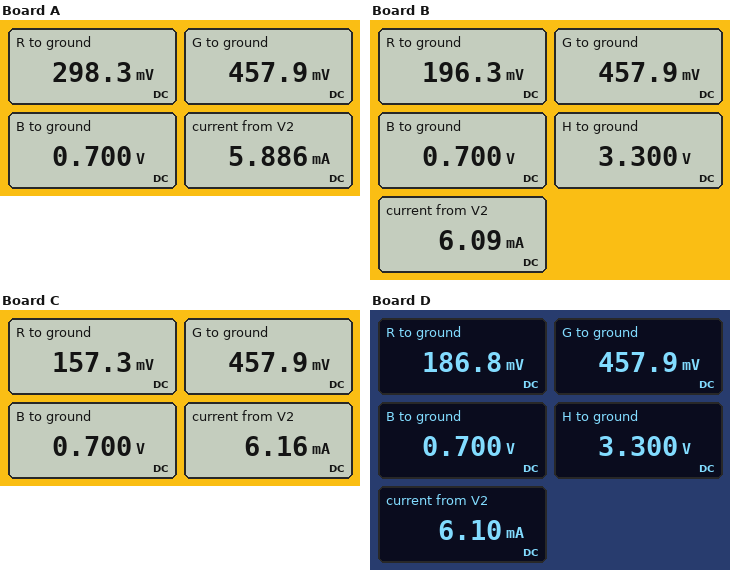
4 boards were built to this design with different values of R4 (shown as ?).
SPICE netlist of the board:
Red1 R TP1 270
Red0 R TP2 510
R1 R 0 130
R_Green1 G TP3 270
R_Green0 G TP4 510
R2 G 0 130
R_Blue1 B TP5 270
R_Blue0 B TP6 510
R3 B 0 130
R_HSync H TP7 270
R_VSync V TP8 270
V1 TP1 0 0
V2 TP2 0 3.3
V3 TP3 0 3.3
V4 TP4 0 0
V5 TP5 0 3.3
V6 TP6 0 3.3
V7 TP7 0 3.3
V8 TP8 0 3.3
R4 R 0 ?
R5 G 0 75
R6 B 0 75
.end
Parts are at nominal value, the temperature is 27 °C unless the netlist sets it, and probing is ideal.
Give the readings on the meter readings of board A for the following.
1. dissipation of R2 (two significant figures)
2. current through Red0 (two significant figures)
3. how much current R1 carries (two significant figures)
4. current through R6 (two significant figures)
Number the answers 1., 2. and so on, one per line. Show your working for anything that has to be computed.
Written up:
1. (457.9 mV)^2 / 130 Ω = 1.6 mW
2. (3.3 V - 298.3 mV) / 510 Ω = 5.9 mA
3. (298.3 mV) / 130 Ω = 2.3 mA
4. (700 mV) / 75 Ω = 9.3 mA
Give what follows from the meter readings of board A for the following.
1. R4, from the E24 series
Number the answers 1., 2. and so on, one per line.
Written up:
1. 120 Ω
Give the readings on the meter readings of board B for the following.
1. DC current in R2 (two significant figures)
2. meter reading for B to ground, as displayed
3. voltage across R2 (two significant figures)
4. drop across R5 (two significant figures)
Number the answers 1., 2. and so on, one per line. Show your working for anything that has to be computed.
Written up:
1. (457.9 mV) / 130 Ω = 3.5 mA
2. 0.700 V
3. 457.9 mV = 460 mV
4. 457.9 mV = 460 mV
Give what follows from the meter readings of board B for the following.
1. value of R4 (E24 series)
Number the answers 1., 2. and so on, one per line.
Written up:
1. 51 Ω
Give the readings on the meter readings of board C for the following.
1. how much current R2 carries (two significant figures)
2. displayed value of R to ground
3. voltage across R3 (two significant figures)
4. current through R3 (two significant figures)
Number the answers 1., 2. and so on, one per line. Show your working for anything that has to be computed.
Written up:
1. (457.9 mV) / 130 Ω = 3.5 mA
2. 157.3 mV
3. 700 mV = 700 mV
4. (700 mV) / 130 Ω = 5.4 mA
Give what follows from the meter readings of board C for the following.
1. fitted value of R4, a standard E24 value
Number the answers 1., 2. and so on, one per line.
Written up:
1. 36 Ω
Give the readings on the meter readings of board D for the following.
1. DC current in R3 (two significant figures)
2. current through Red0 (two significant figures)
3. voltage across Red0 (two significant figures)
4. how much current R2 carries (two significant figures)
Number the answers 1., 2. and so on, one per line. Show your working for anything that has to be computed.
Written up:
1. (700 mV) / 130 Ω = 5.4 mA
2. (3.3 V - 186.8 mV) / 510 Ω = 6.1 mA
3. 3.3 V - 186.8 mV = 3.1 V
4. (457.9 mV) / 130 Ω = 3.5 mA
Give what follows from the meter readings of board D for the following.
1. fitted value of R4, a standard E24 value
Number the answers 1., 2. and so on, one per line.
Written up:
1. 47 Ω
